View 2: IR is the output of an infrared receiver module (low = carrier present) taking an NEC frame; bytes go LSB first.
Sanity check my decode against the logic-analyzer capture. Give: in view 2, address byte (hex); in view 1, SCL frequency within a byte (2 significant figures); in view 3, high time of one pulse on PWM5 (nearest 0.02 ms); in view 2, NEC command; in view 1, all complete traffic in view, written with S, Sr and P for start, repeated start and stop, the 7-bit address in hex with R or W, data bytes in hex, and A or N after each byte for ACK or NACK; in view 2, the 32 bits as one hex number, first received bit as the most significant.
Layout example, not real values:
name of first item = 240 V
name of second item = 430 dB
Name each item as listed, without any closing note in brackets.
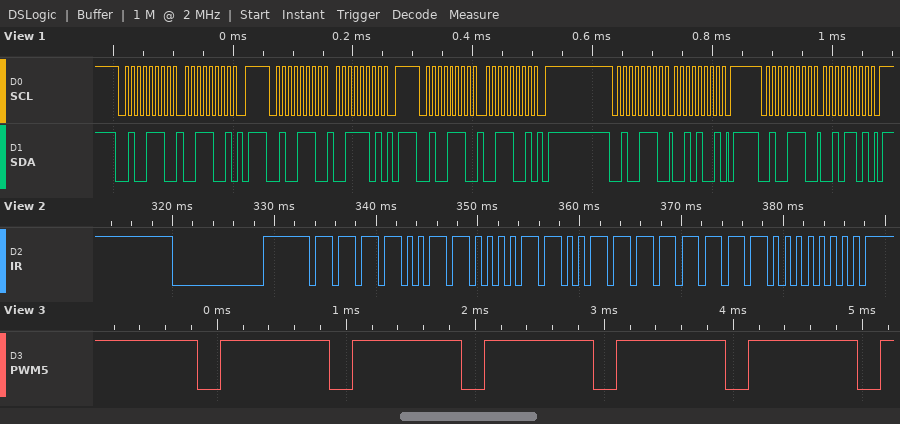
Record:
in view 2, address byte = 0xCF
in view 1, SCL frequency within a byte = 100 kHz
in view 3, high time of one pulse on PWM5 = 0.84 ms
in view 2, NEC command = 0xFF
in view 1, all complete traffic in view, written with S, Sr and P for start, repeated start and stop, the 7-bit address in hex with R or W, data bytes in hex, and A or N after each byte for ACK or NACK = S 27W A 39 A P S 27W A 3D A P S 27W A 39 A P S 27W A 29 A P S 27W A 2D A P
in view 2, the 32 bits as one hex number, first received bit as the most significant = 0xF30CFF00
